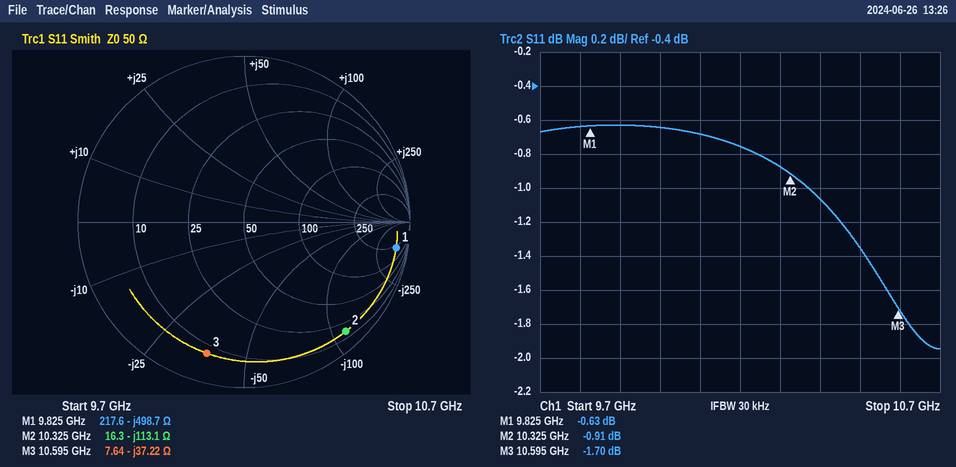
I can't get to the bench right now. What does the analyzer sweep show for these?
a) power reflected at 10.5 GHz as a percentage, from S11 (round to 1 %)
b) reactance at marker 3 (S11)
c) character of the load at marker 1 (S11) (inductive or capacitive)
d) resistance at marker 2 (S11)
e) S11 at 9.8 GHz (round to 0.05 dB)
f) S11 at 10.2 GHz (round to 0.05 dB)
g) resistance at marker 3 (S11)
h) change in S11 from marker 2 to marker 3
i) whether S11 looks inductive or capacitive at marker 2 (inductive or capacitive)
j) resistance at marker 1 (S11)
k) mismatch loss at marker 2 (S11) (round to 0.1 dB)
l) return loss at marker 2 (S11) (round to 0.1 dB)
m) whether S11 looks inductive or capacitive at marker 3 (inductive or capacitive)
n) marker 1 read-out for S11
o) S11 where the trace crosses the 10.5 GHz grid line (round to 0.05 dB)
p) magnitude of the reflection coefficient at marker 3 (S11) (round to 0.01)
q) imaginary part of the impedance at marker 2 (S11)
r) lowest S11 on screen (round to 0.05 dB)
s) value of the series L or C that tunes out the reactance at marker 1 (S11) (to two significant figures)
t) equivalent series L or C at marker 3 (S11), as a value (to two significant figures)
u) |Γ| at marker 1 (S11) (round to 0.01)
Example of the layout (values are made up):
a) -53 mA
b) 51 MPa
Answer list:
a) 73 %
b) -37.22 Ω
c) capacitive
d) 16.3 Ω
e) -0.65 dB
f) -0.75 dB
g) 7.64 Ω
h) -0.79 dB
i) capacitive
j) 217.6 Ω
k) 7.2 dB
l) 0.9 dB
m) capacitive
n) -0.63 dB
o) -1.35 dB
p) 0.82
q) -113.1 Ω
r) -1.95 dB
s) 8.1 nH
t) 400 fF
u) 0.93
